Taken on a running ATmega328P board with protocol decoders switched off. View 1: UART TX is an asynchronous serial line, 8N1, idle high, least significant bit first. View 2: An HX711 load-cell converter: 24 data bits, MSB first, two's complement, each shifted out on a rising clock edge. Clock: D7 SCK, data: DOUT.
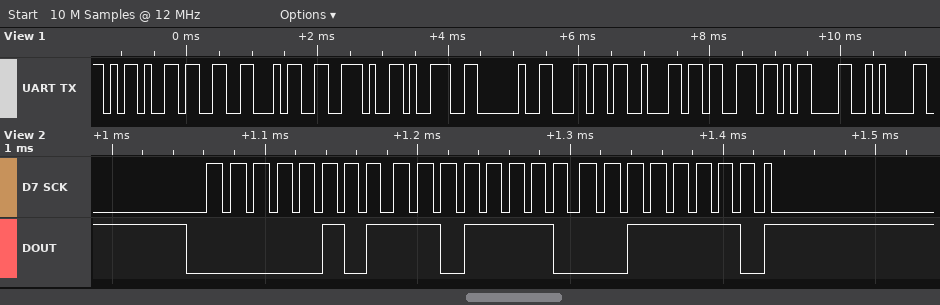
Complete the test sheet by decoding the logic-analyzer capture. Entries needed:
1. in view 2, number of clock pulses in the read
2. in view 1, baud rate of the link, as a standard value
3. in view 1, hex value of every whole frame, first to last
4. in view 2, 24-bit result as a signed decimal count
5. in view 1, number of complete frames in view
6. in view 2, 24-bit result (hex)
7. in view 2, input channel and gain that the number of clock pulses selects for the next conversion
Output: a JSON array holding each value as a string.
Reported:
["25", "9600 baud", "2D 33 34 2E 39 20 6C 62 73 0D 0A", "384574", "11", "0x05DE3E", "channel A, gain 128"]
